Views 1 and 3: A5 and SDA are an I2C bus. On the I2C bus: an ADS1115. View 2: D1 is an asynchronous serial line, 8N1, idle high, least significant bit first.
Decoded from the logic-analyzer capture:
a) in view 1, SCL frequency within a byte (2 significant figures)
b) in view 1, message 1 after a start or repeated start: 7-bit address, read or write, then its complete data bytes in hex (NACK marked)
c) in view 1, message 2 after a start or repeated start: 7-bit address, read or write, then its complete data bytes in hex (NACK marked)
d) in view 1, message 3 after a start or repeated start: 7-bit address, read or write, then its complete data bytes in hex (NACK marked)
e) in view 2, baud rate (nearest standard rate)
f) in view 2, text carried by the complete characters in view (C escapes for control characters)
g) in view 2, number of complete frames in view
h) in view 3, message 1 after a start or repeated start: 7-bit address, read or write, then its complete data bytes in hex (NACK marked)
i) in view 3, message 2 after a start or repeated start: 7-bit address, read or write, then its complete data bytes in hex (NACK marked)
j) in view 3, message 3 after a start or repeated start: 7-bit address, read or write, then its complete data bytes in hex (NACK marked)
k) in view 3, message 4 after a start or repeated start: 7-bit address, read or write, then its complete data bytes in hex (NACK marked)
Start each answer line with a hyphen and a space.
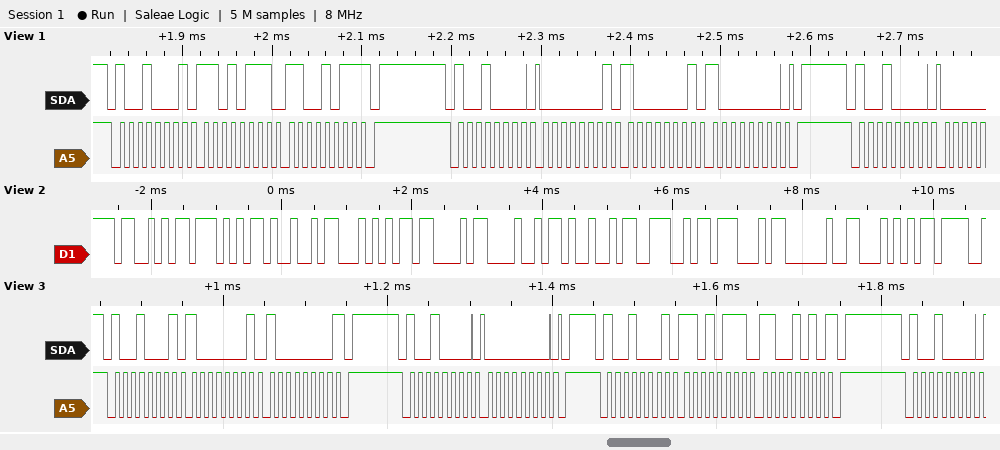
- 100 kHz
- 0x48 read: D7 CB NACK
- 0x48 write: 01 81 80
- 0x48 write
- 9600 baud
- "SWITCHING T"
- 11
- 0x48 read: 81 80 NACK
- 0x48 write: 00
- 0x48 read: D7 CA NACK
- 0x48 write
